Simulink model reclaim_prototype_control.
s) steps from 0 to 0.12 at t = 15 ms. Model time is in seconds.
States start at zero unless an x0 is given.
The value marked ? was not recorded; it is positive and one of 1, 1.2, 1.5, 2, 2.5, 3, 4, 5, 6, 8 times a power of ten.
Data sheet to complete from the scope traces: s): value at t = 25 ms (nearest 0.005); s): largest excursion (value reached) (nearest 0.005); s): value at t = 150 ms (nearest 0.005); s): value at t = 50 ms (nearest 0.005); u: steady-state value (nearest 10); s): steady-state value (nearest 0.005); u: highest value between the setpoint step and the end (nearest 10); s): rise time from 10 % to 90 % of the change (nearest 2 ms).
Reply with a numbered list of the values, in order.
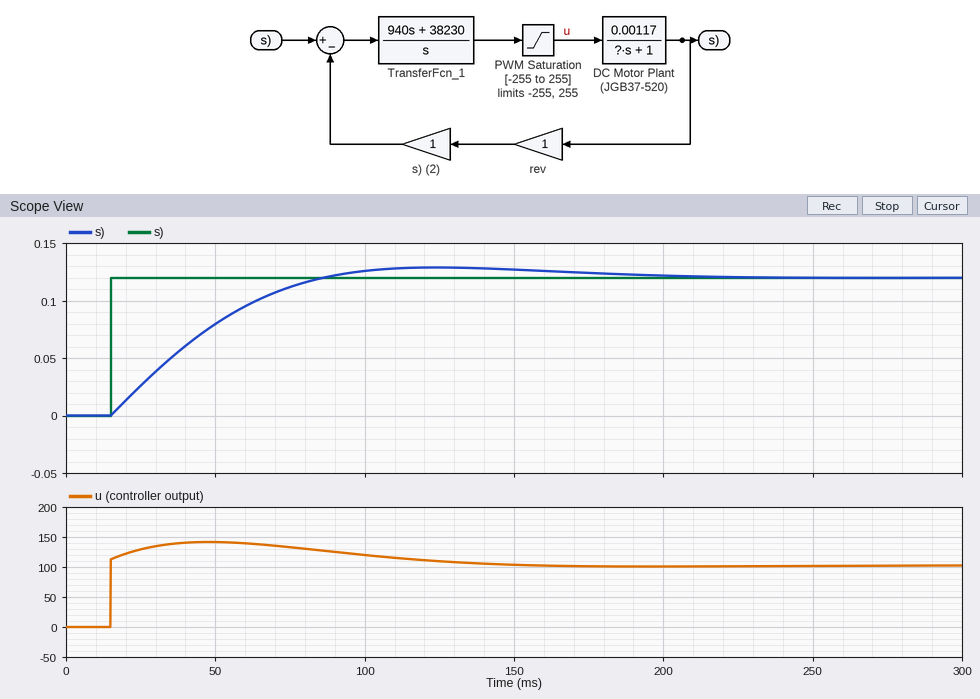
1. 0.025
2. 0.130
3. 0.125
4. 0.080
5. 100
6. 0.120
7. 140
8. 52 ms
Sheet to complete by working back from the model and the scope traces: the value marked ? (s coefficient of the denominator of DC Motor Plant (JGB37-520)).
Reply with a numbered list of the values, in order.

1. 0.05
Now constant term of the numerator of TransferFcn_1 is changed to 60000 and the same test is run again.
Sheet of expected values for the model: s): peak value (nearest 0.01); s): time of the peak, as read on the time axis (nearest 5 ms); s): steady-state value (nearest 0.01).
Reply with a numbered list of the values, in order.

1. 0.14
2. 95 ms
3. 0.12
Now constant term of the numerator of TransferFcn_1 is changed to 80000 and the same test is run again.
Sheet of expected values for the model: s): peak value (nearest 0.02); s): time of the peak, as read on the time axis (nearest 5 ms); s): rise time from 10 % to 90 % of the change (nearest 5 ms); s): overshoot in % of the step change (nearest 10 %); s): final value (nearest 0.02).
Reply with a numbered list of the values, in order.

1. 0.14
2. 85 ms
3. 30 ms
4. 20 %
5. 0.12
